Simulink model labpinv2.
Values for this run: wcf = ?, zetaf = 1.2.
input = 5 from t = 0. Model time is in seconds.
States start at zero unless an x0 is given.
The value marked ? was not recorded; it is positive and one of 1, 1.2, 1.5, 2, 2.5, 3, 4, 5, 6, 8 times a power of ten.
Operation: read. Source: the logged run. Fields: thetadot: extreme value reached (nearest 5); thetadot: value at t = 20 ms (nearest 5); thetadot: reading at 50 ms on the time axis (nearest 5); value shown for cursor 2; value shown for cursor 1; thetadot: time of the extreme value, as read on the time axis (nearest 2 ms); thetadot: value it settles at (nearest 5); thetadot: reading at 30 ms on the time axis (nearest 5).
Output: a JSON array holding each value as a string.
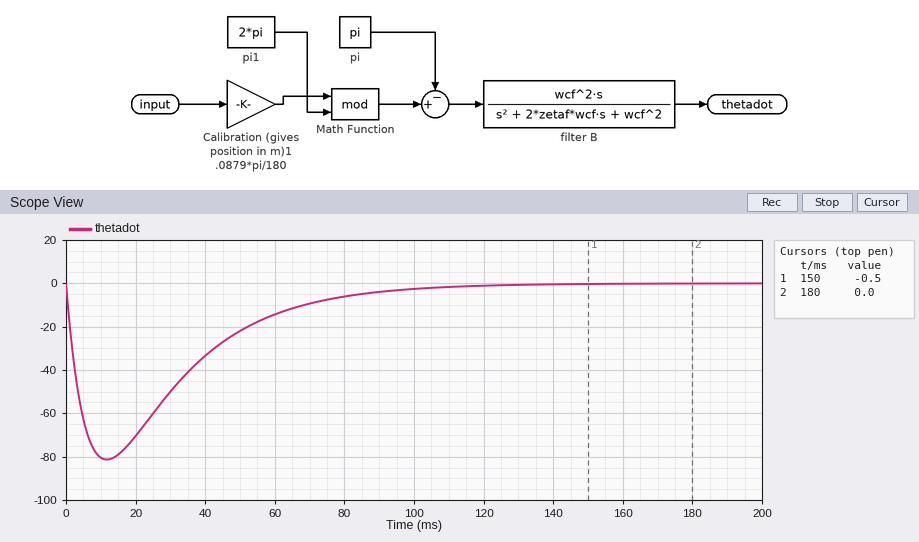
["-80", "-70", "-20", "0.0", "-0.5", "12 ms", "0", "-50"]
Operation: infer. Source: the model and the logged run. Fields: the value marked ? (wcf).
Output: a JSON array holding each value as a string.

["80"]
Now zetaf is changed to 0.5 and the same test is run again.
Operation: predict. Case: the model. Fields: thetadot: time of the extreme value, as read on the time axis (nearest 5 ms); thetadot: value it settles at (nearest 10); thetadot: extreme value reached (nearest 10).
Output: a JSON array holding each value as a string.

["15 ms", "0", "-140"]
